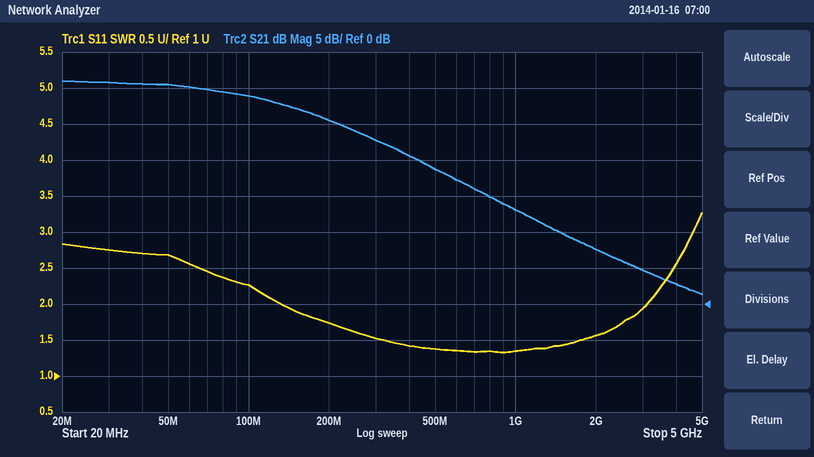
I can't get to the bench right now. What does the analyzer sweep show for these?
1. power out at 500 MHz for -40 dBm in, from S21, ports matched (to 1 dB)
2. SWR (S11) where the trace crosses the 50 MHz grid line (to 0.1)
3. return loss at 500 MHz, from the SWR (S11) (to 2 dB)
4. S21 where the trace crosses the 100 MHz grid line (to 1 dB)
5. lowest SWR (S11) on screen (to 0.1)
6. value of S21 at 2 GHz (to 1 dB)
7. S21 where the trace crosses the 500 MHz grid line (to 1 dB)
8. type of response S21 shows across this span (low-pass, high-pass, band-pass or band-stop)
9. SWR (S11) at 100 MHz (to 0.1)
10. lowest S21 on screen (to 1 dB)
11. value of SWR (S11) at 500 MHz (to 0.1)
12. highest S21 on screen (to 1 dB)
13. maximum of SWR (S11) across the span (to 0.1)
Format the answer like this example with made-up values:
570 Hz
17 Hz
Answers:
-21 dBm
2.7
16 dB
29 dB
1.3
8 dB
19 dB
low-pass
2.3
1 dB
1.4
31 dB
3.3
